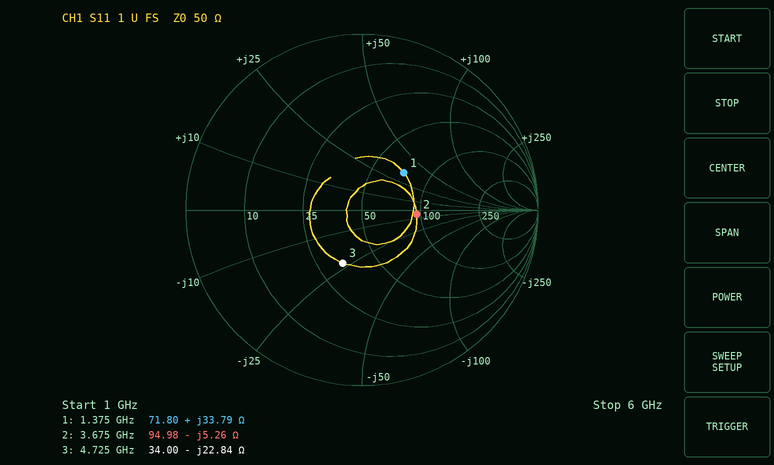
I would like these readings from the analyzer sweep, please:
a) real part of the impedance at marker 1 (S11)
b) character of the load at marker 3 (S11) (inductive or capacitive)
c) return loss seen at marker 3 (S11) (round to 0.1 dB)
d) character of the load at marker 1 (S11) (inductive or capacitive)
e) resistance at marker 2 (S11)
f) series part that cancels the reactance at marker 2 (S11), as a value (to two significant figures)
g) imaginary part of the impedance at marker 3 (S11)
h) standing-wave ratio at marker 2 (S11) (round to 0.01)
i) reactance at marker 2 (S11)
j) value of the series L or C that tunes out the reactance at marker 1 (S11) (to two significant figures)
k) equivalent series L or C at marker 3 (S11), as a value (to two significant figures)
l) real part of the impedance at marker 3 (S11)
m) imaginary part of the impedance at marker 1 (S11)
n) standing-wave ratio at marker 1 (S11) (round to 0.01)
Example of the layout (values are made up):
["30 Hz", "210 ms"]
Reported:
["71.80 Ω", "capacitive", "9.9 dB", "inductive", "94.98 Ω", "230 pH", "-22.84 Ω", "1.91", "-5.26 Ω", "3.4 pF", "1.5 pF", "34.00 Ω", "+33.79 Ω", "1.93"]
